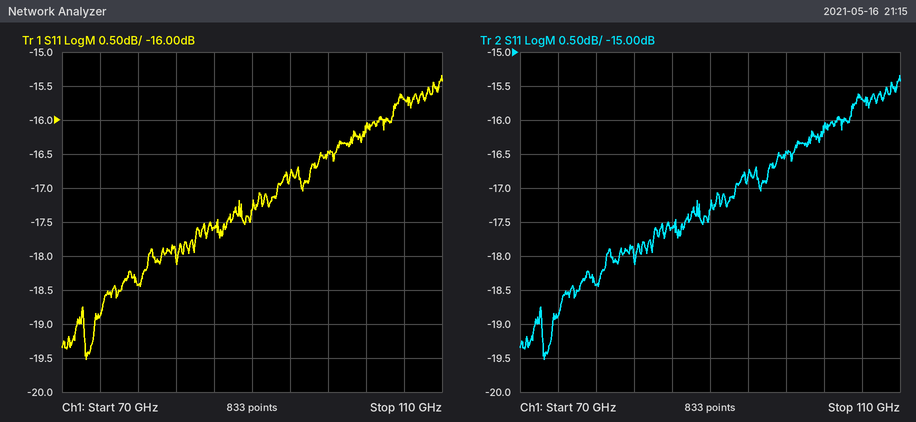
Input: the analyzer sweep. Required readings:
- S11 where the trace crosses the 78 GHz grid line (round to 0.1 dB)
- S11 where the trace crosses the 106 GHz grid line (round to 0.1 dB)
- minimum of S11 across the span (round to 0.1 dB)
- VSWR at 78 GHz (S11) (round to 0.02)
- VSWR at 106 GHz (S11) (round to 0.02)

-18.4 dB
-15.7 dB
-19.5 dB
1.28
1.40
